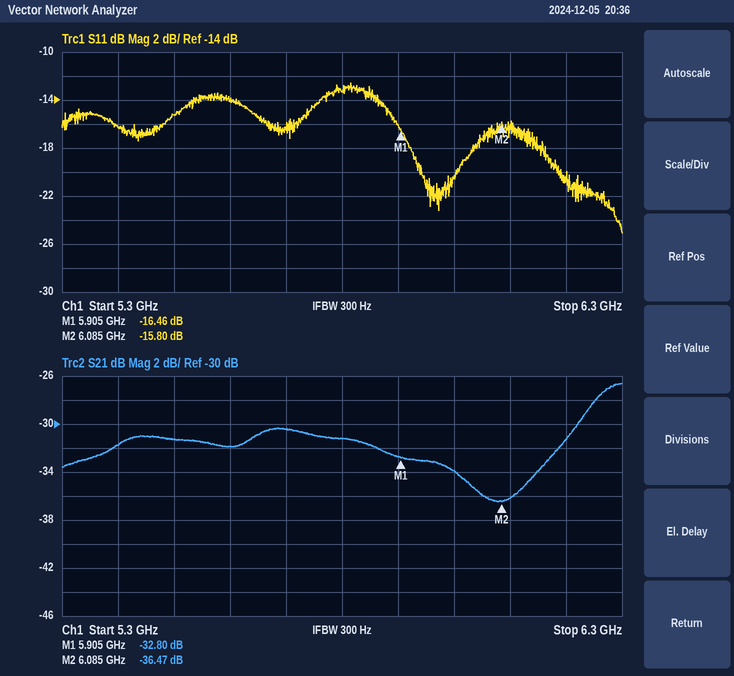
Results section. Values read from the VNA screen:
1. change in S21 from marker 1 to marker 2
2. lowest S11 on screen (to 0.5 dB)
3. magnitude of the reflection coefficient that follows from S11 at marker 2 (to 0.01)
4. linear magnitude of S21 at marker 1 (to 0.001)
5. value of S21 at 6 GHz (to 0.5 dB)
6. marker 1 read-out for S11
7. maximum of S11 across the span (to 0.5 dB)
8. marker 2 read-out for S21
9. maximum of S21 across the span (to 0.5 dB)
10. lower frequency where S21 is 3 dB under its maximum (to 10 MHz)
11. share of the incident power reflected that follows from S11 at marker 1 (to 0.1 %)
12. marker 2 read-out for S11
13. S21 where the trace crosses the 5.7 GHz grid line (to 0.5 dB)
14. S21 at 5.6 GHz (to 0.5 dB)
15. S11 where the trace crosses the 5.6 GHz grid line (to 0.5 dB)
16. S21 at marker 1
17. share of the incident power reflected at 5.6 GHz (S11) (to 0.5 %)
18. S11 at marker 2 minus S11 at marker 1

-3.67 dB
-25.0 dB
0.16
0.023
-34.0 dB
-16.46 dB
-12.5 dB
-36.47 dB
-26.5 dB
6.23 GHz
2.3 %
-15.80 dB
-30.5 dB
-32.0 dB
-14.0 dB
-32.80 dB
4.0 %
0.66 dB
